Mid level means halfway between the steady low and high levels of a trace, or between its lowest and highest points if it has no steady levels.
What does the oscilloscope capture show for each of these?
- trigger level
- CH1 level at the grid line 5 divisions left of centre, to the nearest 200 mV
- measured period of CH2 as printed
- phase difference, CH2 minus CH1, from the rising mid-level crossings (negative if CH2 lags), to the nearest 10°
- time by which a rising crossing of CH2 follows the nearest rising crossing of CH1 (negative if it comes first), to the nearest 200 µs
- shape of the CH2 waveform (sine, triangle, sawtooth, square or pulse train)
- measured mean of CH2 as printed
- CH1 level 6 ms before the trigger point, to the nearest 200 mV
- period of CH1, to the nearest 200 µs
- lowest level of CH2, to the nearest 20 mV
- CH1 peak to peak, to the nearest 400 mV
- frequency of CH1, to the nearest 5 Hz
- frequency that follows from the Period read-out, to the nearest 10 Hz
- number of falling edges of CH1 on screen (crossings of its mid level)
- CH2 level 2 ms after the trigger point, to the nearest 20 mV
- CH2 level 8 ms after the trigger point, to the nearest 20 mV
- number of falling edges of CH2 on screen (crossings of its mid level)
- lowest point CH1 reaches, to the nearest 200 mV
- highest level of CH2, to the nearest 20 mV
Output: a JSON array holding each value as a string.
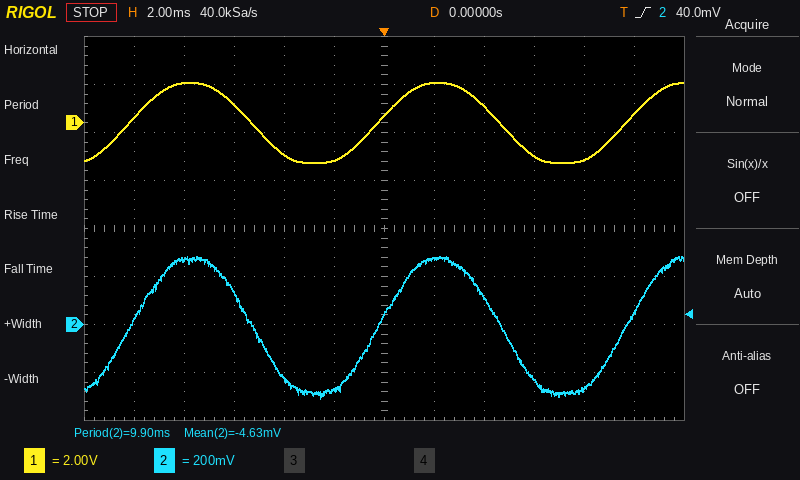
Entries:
["40.0 mV", "200 mV", "9.90 ms", "0°", "0.0 ms", "sine", "-4.63 mV", "800 mV", "10.0 ms", "-300 mV", "3.2 V", "100 Hz", "100 Hz", "2", "280 mV", "-260 mV", "2", "-1.6 V", "280 mV"]
